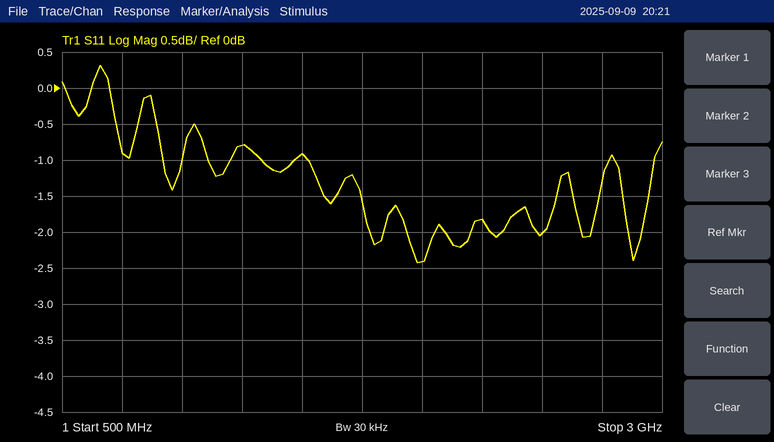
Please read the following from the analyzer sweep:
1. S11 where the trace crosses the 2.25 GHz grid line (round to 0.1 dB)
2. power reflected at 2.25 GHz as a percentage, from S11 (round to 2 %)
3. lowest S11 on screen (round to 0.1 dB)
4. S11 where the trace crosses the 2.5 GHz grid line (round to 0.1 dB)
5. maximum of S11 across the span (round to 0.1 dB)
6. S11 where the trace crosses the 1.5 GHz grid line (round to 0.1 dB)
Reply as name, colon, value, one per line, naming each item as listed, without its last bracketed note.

S11 where the trace crosses the 2.25 GHz grid line: -1.8 dB
power reflected at 2.25 GHz as a percentage, from S11: 66 %
lowest S11 on screen: -2.4 dB
S11 where the trace crosses the 2.5 GHz grid line: -2.0 dB
maximum of S11 across the span: 0.3 dB
S11 where the trace crosses the 1.5 GHz grid line: -0.9 dB
